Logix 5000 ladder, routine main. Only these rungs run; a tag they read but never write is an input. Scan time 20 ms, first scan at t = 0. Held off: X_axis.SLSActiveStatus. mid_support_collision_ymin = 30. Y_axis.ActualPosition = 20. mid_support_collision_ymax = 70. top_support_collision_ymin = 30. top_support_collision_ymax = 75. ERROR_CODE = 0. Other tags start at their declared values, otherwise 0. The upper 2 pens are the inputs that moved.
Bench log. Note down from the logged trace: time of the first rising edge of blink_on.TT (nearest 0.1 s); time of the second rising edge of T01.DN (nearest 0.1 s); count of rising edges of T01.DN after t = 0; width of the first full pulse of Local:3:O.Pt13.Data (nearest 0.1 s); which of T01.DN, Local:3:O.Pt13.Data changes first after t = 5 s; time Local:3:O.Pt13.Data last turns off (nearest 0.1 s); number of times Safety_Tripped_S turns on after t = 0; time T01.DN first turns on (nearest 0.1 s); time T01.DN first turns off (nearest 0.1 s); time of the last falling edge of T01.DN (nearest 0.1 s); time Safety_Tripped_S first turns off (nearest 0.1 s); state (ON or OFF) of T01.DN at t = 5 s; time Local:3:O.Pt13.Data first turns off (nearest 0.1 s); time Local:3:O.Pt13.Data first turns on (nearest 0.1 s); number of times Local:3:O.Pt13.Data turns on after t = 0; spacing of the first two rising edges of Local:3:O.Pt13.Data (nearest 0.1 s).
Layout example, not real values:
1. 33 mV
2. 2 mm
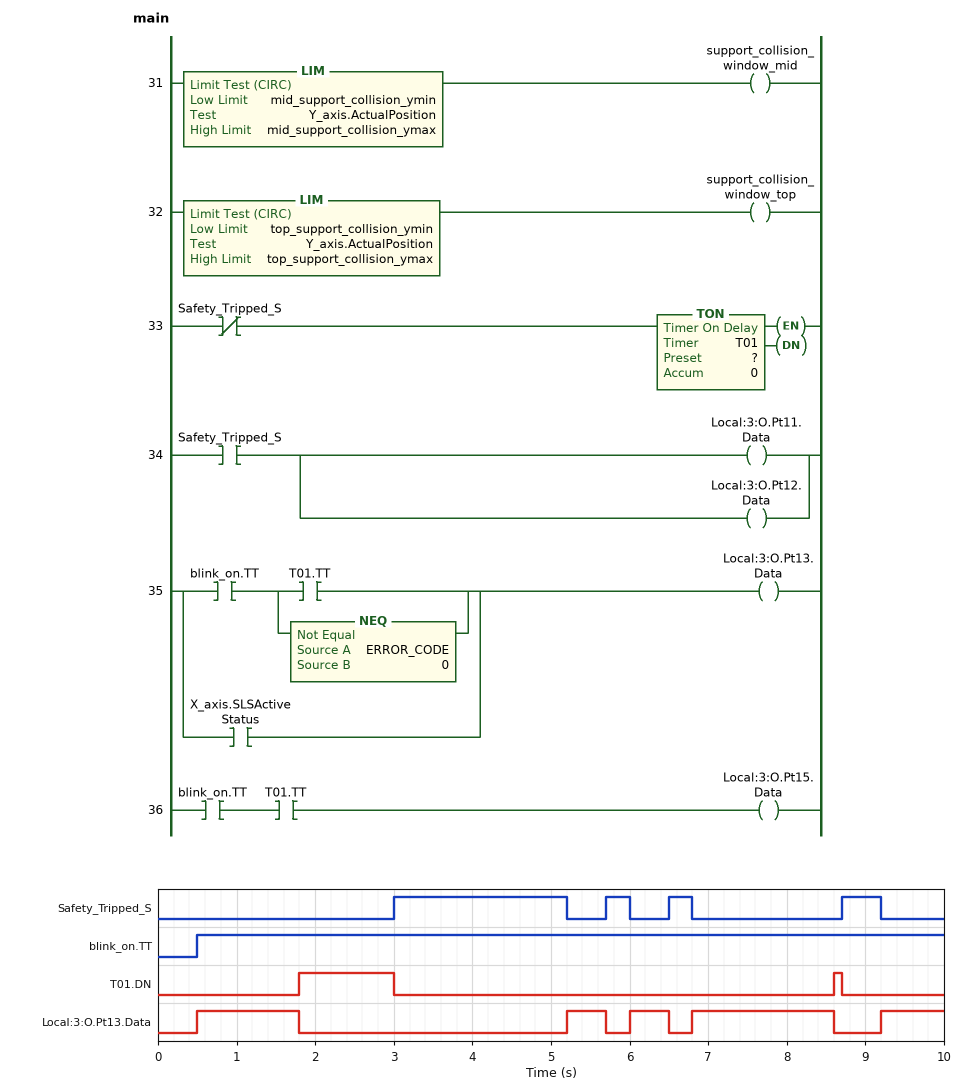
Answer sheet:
1. 0.5 s
2. 8.6 s
3. 2
4. 1.3 s
5. Local:3:O.Pt13.Data
6. 8.6 s
7. 4
8. 1.8 s
9. 3.0 s
10. 8.7 s
11. 5.2 s
12. OFF
13. 1.8 s
14. 0.5 s
15. 5
16. 4.7 s
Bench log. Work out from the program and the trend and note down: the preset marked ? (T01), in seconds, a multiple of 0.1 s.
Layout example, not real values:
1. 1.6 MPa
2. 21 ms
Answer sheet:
1. 1.8 s
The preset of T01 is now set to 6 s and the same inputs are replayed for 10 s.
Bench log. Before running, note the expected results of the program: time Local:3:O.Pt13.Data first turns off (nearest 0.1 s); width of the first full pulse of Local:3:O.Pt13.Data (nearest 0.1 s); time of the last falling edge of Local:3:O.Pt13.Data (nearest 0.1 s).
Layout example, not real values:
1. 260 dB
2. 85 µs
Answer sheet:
1. 3.0 s
2. 2.5 s
3. 8.7 s
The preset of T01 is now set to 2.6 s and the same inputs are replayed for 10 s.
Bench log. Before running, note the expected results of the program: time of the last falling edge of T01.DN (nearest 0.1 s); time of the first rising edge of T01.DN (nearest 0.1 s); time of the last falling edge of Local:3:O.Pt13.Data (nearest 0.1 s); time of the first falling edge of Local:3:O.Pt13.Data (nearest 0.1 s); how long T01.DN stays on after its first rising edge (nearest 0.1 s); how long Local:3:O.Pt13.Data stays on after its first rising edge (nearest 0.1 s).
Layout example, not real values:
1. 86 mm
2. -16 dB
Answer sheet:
1. 3.0 s
2. 2.6 s
3. 8.7 s
4. 2.6 s
5. 0.4 s
6. 2.1 s
